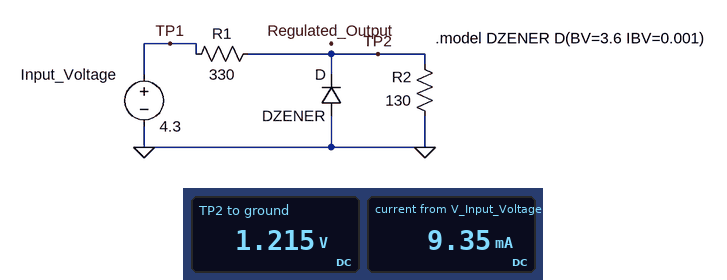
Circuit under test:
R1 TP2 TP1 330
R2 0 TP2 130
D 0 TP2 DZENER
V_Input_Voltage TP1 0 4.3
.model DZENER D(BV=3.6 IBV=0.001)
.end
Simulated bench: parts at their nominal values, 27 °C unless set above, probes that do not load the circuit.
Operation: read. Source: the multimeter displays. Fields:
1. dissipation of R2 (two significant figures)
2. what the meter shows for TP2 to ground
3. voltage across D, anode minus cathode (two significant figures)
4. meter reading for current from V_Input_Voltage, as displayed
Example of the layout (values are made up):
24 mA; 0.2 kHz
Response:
11 mW; 1.215 V; -1.2 V; 9.35 mA
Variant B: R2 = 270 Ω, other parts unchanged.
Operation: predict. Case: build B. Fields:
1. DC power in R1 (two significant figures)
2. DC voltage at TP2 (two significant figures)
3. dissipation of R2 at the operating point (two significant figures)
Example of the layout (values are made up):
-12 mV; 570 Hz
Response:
17 mW; 1.9 V; 14 mW
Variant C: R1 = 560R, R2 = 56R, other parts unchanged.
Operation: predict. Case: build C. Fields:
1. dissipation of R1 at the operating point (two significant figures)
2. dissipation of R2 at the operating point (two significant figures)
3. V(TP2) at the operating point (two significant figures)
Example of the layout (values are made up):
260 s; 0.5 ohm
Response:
27 mW; 2.7 mW; 390 mV
